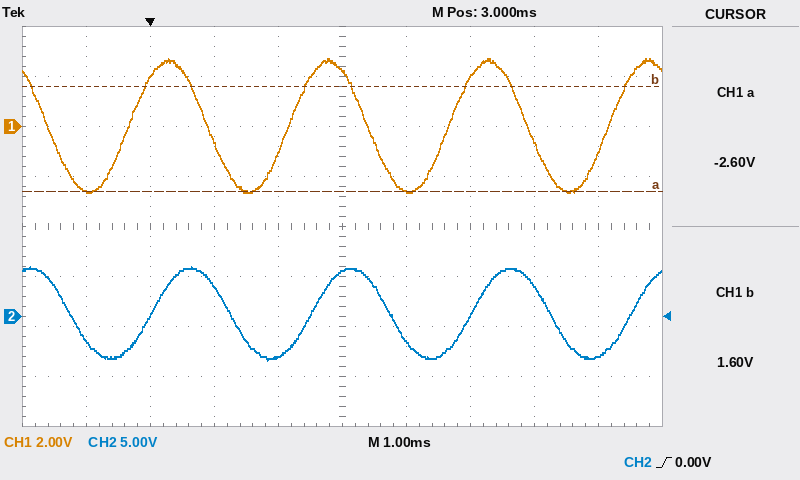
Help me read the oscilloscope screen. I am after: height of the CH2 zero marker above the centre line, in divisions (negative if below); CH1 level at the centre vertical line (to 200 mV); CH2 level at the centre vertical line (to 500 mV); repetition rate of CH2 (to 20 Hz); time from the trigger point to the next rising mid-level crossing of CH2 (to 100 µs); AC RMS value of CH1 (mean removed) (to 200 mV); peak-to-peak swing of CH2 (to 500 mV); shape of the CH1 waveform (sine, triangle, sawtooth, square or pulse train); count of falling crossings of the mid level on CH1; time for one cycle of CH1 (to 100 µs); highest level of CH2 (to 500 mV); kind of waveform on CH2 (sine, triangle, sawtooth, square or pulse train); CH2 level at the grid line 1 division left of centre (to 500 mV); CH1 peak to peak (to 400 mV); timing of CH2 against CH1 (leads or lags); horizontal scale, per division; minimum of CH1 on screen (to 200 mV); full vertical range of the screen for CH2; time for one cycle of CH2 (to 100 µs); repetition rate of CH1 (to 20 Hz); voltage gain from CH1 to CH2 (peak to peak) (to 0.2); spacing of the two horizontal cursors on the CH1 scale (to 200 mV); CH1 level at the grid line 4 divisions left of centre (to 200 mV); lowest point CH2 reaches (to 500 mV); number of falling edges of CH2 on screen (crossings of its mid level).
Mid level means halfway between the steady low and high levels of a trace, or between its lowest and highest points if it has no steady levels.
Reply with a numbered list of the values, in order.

1. -1.8 div
2. 2.2 V
3. 4.5 V
4. 400 Hz
5. 2.5 ms
6. 1.8 V
7. 9.5 V
8. sine
9. 4
10. 2.5 ms
11. 5.0 V
12. sine
13. -4.0 V
14. 5.2 V
15. lags
16. 1 ms
17. -2.6 V
18. 40 V
19. 2.5 ms
20. 400 Hz
21. 1.8
22. 4.2 V
23. -2.6 V
24. -4.5 V
25. 4
